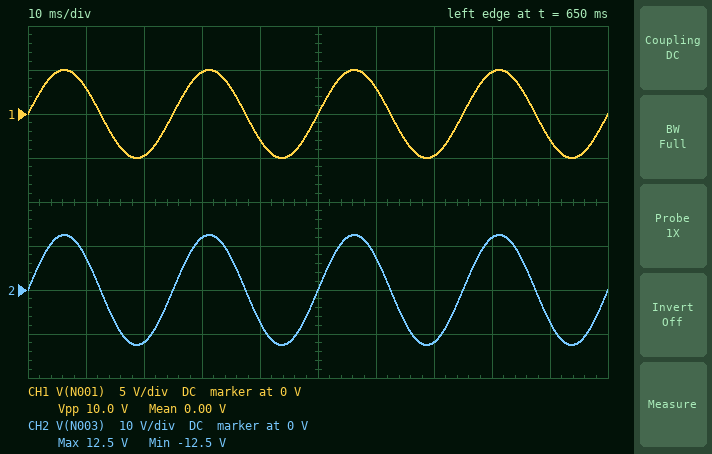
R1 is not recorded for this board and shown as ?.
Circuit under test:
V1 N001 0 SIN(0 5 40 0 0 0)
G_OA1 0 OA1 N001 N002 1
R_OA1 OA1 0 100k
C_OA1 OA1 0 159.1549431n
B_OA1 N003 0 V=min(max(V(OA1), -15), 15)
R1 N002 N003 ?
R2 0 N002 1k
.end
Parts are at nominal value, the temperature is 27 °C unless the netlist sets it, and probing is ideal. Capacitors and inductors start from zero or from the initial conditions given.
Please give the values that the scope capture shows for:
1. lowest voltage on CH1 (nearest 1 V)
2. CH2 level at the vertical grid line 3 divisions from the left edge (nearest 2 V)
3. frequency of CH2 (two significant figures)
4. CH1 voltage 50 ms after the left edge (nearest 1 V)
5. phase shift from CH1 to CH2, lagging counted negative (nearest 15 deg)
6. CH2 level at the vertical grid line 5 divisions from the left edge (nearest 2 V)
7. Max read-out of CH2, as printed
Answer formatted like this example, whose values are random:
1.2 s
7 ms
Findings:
-5 V
12 V
40 Hz
0 V
0 deg
0 V
12.5 V
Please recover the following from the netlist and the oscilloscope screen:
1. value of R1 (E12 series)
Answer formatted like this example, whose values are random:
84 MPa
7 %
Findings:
1.5 kΩ
